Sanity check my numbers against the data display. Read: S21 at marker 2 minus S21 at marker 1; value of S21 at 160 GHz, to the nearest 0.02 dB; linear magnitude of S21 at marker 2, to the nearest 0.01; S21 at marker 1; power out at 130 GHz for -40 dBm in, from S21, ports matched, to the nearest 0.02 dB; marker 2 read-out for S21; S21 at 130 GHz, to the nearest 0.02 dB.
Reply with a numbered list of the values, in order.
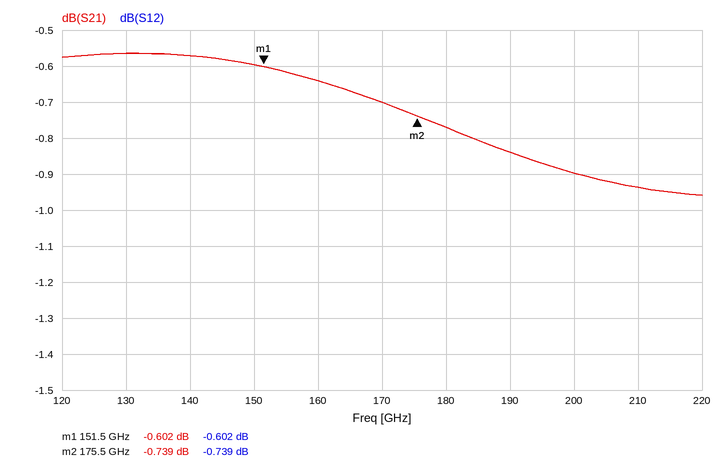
1. -0.137 dB
2. -0.64 dB
3. 0.92
4. -0.602 dB
5. -40.56 dBm
6. -0.739 dB
7. -0.56 dB
